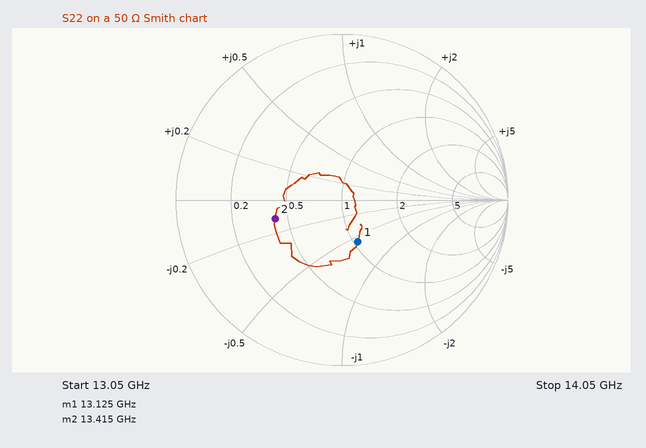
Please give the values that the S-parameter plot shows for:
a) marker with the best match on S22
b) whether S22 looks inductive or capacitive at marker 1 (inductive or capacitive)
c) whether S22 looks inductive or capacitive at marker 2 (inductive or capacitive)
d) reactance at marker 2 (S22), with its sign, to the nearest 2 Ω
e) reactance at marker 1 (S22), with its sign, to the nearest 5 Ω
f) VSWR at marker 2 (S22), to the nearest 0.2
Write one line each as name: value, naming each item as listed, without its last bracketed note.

marker with the best match on S22: marker 1
whether S22 looks inductive or capacitive at marker 1: capacitive
whether S22 looks inductive or capacitive at marker 2: capacitive
reactance at marker 2 (S22), with its sign, to the nearest 2 Ω: -6 Ω
reactance at marker 1 (S22), with its sign, to the nearest 5 Ω: -30 Ω
VSWR at marker 2 (S22), to the nearest 0.2: 2.4
